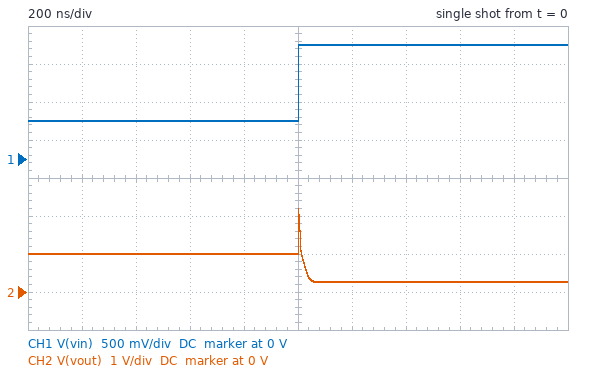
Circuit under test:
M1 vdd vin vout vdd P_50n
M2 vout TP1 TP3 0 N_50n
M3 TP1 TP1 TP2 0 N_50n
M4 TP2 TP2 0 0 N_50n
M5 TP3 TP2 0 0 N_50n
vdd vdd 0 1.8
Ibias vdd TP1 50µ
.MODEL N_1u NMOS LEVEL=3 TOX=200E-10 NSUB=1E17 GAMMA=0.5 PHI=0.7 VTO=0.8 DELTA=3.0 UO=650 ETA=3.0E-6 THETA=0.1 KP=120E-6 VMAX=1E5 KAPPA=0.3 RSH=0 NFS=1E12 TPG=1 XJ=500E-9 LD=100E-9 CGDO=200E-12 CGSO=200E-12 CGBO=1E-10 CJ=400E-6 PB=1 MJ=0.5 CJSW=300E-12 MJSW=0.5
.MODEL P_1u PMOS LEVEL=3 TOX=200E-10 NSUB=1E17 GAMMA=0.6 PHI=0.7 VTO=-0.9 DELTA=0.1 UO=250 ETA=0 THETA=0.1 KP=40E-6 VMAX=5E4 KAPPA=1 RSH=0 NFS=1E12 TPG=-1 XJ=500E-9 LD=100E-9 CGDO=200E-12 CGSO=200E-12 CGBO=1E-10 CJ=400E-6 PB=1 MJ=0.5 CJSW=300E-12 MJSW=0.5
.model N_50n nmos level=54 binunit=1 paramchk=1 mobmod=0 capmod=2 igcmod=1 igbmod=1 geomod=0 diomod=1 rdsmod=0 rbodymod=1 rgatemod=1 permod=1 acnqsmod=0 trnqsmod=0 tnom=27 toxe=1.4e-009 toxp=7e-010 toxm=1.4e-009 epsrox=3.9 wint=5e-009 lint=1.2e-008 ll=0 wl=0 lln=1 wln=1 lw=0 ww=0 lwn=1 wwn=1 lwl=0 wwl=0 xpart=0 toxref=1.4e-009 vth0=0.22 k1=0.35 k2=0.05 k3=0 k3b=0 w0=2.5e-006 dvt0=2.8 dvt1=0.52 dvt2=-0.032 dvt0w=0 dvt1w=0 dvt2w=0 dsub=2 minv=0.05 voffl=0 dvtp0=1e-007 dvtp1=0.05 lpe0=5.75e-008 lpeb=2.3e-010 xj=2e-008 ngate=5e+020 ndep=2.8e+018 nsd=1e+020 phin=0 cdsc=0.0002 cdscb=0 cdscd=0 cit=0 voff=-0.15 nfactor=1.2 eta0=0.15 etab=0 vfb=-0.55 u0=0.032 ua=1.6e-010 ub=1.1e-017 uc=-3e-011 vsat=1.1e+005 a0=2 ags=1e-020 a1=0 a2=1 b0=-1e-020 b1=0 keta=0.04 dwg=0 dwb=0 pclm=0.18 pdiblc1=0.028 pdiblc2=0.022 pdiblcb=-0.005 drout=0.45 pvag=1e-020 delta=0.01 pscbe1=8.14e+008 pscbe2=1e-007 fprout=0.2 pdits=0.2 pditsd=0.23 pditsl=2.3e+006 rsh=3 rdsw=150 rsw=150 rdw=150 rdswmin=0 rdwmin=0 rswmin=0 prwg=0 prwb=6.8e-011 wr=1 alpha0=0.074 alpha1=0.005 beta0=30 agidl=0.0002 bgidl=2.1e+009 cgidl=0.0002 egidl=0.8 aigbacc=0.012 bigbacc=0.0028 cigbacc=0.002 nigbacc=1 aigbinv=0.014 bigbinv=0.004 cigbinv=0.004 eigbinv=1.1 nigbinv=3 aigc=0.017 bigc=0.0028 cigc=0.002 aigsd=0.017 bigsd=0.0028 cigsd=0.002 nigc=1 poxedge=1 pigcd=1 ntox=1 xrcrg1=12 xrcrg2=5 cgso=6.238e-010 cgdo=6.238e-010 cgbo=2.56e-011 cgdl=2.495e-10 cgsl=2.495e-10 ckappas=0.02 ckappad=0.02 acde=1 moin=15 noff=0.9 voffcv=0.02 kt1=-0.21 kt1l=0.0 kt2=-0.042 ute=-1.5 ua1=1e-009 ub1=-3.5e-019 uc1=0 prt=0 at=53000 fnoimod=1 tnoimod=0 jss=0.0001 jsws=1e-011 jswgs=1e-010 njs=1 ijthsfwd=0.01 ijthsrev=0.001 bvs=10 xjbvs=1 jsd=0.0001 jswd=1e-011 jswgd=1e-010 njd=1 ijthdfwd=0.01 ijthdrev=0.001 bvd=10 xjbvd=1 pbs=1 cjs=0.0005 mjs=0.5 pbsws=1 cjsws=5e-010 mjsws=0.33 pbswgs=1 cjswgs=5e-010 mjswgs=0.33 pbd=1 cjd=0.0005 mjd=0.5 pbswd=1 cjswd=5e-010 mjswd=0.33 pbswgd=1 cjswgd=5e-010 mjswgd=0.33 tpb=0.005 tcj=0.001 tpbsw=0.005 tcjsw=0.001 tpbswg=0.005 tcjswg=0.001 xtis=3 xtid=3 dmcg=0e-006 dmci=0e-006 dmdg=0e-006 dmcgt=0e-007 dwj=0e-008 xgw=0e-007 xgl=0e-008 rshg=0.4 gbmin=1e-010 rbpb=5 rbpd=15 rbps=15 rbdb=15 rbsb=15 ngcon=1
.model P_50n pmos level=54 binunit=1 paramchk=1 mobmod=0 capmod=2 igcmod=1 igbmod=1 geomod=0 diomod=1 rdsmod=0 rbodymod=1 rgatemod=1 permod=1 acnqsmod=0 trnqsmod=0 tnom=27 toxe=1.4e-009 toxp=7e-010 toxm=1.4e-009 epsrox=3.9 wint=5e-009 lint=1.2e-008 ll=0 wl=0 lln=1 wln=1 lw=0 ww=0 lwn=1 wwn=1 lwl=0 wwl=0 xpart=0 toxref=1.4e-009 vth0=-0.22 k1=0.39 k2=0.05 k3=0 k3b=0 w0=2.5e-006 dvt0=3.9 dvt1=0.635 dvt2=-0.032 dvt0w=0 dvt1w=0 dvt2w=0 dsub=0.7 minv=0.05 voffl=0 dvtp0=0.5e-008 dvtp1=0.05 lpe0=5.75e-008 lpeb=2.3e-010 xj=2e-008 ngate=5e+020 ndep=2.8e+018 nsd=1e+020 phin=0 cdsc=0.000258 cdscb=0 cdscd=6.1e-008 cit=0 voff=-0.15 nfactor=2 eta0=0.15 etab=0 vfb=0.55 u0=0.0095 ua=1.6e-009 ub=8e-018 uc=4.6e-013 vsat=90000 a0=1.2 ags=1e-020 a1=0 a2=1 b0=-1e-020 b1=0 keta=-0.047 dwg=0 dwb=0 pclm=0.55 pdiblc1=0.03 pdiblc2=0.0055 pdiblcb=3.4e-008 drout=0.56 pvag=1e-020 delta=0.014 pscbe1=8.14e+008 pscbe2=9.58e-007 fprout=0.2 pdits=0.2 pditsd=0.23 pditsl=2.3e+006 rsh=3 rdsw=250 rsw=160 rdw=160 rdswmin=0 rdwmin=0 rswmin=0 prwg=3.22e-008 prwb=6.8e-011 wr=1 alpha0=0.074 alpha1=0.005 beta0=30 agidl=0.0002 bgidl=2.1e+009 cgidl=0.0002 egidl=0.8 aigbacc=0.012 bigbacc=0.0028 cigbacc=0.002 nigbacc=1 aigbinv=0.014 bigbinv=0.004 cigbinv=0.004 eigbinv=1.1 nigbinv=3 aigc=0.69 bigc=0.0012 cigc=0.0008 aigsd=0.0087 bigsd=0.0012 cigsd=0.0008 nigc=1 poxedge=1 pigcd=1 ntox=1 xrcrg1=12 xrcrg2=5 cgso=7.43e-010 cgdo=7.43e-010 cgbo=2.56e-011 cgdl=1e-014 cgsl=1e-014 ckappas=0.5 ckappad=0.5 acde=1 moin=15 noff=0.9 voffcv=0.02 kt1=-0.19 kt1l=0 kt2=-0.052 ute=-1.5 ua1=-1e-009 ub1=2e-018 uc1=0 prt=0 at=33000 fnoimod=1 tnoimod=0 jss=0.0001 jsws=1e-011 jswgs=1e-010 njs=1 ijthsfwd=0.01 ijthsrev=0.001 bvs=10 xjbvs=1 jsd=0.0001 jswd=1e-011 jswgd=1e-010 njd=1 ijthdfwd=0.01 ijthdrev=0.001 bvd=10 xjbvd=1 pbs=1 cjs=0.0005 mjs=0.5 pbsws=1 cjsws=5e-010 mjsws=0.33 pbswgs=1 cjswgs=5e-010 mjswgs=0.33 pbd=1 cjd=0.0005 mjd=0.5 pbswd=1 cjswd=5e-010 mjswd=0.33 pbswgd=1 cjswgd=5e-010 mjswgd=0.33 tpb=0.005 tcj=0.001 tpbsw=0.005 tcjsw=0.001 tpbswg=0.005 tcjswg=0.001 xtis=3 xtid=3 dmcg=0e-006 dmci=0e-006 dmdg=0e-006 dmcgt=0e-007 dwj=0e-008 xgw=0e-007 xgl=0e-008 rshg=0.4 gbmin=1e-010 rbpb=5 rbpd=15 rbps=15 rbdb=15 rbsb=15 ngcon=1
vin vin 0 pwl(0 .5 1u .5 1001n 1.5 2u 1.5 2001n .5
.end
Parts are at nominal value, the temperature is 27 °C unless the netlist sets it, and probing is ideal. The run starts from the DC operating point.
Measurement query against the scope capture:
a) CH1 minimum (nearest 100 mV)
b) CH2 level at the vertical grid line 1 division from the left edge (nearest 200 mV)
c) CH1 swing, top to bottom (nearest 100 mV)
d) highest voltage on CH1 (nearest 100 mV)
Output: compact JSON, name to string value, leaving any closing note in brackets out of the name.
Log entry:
{"CH1 minimum": "500 mV", "CH2 level at the vertical grid line 1 division from the left edge": "1.0 V", "CH1 swing, top to bottom": "1.0 V", "highest voltage on CH1": "1.5 V"}
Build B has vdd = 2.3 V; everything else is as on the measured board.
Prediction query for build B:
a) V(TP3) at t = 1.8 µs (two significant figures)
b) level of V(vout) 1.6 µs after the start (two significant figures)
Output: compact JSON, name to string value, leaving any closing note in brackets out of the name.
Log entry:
{"V(TP3) at t = 1.8 µs": "400 mV", "level of V(vout) 1.6 µs after the start": "580 mV"}
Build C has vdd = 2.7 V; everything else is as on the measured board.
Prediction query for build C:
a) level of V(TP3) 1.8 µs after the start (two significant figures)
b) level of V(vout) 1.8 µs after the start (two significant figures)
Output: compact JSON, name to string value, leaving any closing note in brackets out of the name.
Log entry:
{"level of V(TP3) 1.8 µs after the start": "660 mV", "level of V(vout) 1.8 µs after the start": "970 mV"}
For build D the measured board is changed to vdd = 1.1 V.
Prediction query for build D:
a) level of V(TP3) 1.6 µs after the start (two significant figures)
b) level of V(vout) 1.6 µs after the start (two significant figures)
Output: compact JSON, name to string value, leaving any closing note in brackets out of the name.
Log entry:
{"level of V(TP3) 1.6 µs after the start": "170 mV", "level of V(vout) 1.6 µs after the start": "230 mV"}
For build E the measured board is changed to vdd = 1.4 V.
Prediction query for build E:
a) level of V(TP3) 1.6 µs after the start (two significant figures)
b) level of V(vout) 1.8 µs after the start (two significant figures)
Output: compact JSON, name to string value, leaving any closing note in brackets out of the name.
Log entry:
{"level of V(TP3) 1.6 µs after the start": "170 mV", "level of V(vout) 1.8 µs after the start": "230 mV"}
